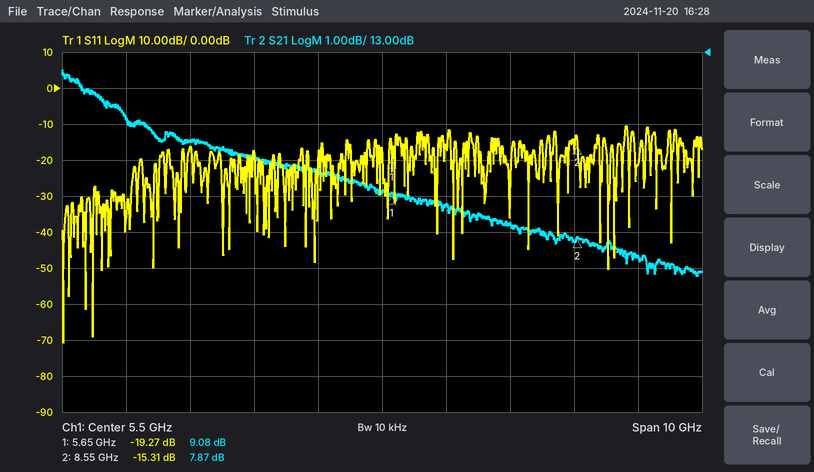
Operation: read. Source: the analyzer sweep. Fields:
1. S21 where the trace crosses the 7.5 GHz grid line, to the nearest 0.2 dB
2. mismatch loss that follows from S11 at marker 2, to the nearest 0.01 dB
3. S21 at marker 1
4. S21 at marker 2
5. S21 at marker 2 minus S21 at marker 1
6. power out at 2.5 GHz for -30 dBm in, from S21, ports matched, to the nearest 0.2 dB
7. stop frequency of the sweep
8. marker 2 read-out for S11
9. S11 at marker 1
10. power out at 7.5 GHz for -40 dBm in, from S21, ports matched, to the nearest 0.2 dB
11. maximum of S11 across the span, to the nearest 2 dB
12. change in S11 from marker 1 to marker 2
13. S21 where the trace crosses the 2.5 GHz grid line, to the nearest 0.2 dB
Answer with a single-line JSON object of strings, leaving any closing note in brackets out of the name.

{"S21 where the trace crosses the 7.5 GHz grid line, to the nearest 0.2 dB": "8.2 dB", "mismatch loss that follows from S11 at marker 2, to the nearest 0.01 dB": "0.13 dB", "S21 at marker 1": "9.08 dB", "S21 at marker 2": "7.87 dB", "S21 at marker 2 minus S21 at marker 1": "-1.21 dB", "power out at 2.5 GHz for -30 dBm in, from S21, ports matched, to the nearest 0.2 dB": "-19.4 dBm", "stop frequency of the sweep": "10.5 GHz", "marker 2 read-out for S11": "-15.31 dB", "S11 at marker 1": "-19.27 dB", "power out at 7.5 GHz for -40 dBm in, from S21, ports matched, to the nearest 0.2 dB": "-31.8 dBm", "maximum of S11 across the span, to the nearest 2 dB": "-10 dB", "change in S11 from marker 1 to marker 2": "3.96 dB", "S21 where the trace crosses the 2.5 GHz grid line, to the nearest 0.2 dB": "10.6 dB"}
